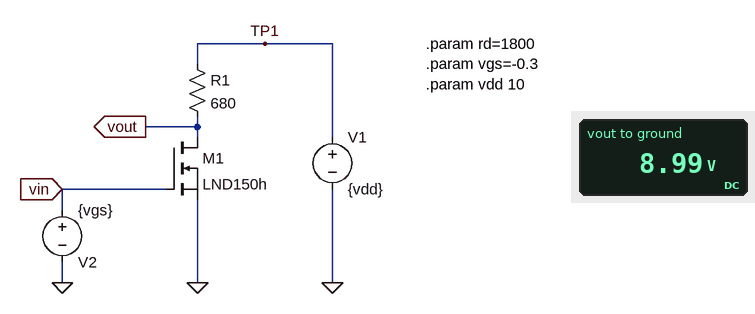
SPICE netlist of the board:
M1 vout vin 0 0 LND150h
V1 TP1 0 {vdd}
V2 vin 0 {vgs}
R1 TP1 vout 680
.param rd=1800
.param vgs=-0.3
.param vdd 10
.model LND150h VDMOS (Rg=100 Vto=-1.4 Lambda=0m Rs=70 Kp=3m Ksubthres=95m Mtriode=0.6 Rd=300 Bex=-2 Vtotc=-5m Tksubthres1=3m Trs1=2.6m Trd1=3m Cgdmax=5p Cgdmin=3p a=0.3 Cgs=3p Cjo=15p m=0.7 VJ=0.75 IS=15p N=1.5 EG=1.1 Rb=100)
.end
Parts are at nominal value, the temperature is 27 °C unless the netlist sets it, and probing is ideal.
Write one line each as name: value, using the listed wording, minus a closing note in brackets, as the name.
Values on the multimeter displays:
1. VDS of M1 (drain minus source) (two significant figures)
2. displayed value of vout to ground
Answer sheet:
VDS of M1 (drain minus source): 9.0 V
displayed value of vout to ground: 8.99 V
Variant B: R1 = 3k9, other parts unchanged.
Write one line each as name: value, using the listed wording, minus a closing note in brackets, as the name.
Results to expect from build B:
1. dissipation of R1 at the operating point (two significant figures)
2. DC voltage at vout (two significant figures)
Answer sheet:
dissipation of R1 at the operating point: 8.6 mW
DC voltage at vout: 4.2 V
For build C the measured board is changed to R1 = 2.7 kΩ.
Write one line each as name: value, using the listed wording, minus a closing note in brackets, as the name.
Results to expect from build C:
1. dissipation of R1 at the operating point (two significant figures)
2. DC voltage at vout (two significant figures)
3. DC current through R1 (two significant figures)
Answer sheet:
dissipation of R1 at the operating point: 6.0 mW
DC voltage at vout: 6.0 V
DC current through R1: 1.5 mA
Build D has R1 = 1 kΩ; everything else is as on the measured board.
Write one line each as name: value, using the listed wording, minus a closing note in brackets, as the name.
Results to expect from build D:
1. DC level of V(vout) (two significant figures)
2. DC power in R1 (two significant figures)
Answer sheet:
DC level of V(vout): 8.5 V
DC power in R1: 2.2 mW
